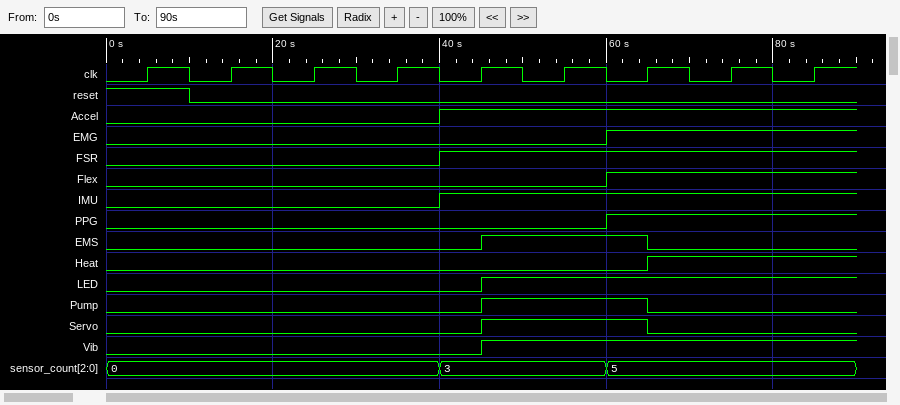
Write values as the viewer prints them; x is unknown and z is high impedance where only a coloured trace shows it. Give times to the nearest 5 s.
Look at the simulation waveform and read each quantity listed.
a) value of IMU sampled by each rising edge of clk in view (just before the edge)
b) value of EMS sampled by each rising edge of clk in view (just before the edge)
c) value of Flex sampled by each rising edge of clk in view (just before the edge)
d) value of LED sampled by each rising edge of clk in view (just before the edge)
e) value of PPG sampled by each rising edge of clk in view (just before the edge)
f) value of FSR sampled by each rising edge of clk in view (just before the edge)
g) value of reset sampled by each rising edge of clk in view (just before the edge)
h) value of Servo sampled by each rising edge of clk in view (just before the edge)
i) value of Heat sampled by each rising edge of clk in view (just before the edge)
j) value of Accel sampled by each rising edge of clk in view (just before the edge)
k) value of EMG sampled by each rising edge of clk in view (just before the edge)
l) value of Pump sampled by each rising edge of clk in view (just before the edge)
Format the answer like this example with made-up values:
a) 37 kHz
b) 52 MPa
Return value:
a) 0 0 0 0 1 1 1 1 1
b) 0 0 0 0 0 1 1 0 0
c) 0 0 0 0 0 0 1 1 1
d) 0 0 0 0 0 1 1 1 1
e) 0 0 0 0 0 0 1 1 1
f) 0 0 0 0 1 1 1 1 1
g) 1 0 0 0 0 0 0 0 0
h) 0 0 0 0 0 1 1 0 0
i) 0 0 0 0 0 0 0 1 1
j) 0 0 0 0 1 1 1 1 1
k) 0 0 0 0 0 0 1 1 1
l) 0 0 0 0 0 1 1 0 0
